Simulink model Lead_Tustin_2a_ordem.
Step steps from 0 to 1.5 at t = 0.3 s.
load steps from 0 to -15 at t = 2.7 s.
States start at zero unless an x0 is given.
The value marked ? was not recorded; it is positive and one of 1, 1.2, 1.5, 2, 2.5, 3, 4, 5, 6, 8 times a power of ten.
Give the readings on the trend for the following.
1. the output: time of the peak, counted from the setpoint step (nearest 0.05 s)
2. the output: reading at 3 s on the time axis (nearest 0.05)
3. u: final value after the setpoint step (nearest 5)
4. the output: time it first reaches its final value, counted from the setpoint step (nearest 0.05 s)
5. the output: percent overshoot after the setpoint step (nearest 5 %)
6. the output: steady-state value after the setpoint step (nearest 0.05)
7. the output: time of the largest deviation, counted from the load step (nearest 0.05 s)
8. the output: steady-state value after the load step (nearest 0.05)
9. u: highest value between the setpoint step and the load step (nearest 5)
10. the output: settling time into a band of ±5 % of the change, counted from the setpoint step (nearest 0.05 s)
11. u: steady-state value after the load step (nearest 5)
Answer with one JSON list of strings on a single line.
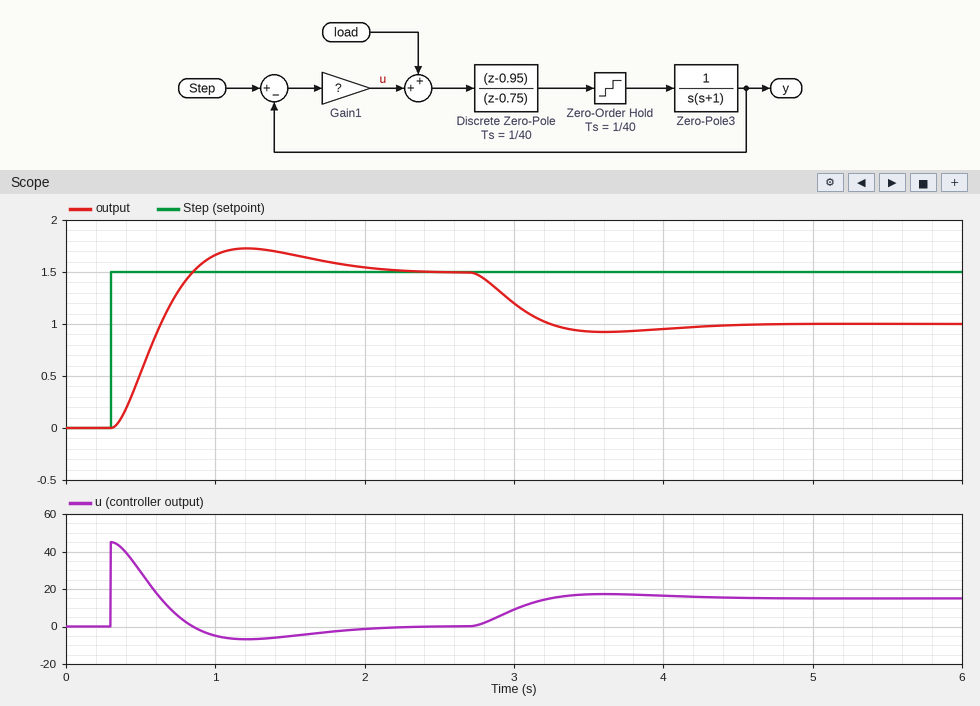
["0.90 s", "1.20", "0", "0.55 s", "15 %", "1.50", "0.90 s", "1.00", "45", "1.55 s", "15"]
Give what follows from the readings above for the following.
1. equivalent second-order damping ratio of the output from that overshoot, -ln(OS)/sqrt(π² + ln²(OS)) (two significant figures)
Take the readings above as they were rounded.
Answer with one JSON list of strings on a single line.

["0.52"]
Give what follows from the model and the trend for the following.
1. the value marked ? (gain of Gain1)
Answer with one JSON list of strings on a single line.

["30"]
